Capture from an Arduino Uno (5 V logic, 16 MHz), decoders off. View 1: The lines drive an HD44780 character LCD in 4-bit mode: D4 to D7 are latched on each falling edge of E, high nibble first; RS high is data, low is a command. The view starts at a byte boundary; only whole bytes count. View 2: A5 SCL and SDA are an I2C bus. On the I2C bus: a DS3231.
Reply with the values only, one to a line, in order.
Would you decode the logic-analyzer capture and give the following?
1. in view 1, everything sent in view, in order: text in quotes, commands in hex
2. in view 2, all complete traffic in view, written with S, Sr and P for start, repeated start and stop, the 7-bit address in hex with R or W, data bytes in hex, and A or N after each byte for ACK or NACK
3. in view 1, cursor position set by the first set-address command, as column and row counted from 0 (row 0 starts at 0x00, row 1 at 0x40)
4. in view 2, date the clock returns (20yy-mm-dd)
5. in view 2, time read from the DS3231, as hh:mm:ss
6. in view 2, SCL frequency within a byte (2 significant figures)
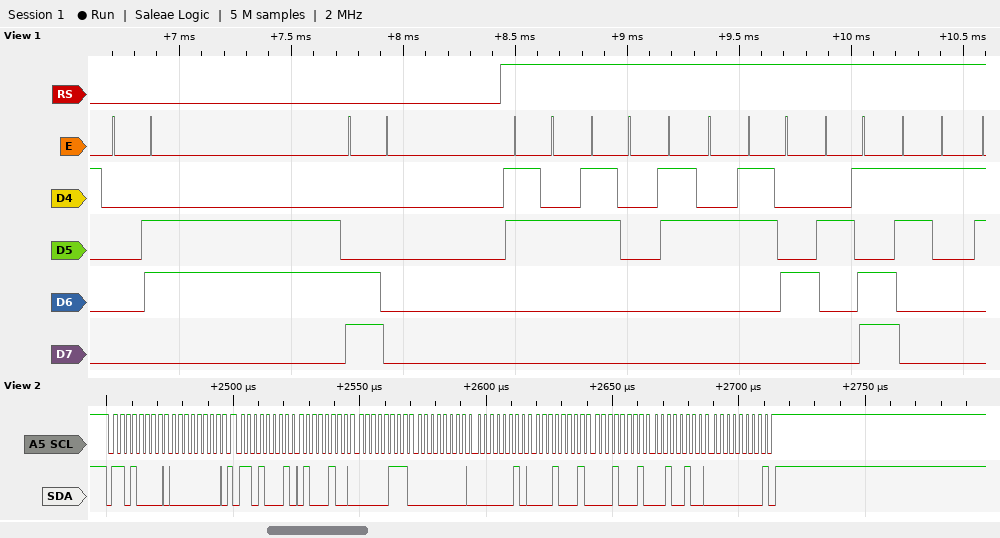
0x06 0xC0 "2024-1"
S 68W A 00 A Sr 68R A 44 A 07 A 00 A 02 A 11 A 11 A 24 A 00 N P
column 0, row 1
2024-11-11
00:07:44
400 kHz
